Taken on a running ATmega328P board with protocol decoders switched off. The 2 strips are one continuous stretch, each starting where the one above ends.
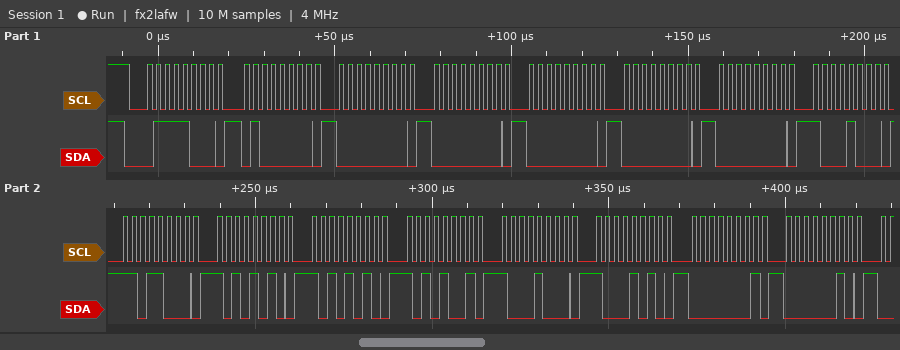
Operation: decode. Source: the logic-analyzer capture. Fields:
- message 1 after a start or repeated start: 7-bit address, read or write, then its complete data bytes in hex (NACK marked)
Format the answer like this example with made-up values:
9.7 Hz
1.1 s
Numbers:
0x3C write: 40 00 00 00 00 00 88 D8 AA AA A9 88 8A 01 02
